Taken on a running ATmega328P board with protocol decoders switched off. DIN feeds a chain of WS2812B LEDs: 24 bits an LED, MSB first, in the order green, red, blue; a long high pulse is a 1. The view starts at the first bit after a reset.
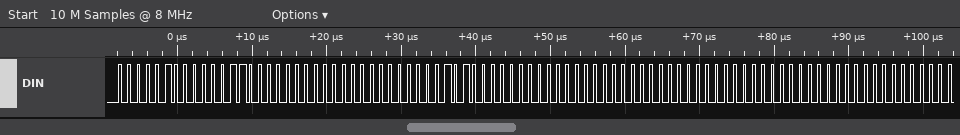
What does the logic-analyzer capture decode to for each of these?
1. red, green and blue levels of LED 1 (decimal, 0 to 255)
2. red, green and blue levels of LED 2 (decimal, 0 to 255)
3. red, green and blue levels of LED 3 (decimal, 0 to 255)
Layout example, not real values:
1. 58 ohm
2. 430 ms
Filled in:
1. 12, 4, 0
2. 20, 0, 0
3. 0, 0, 0
